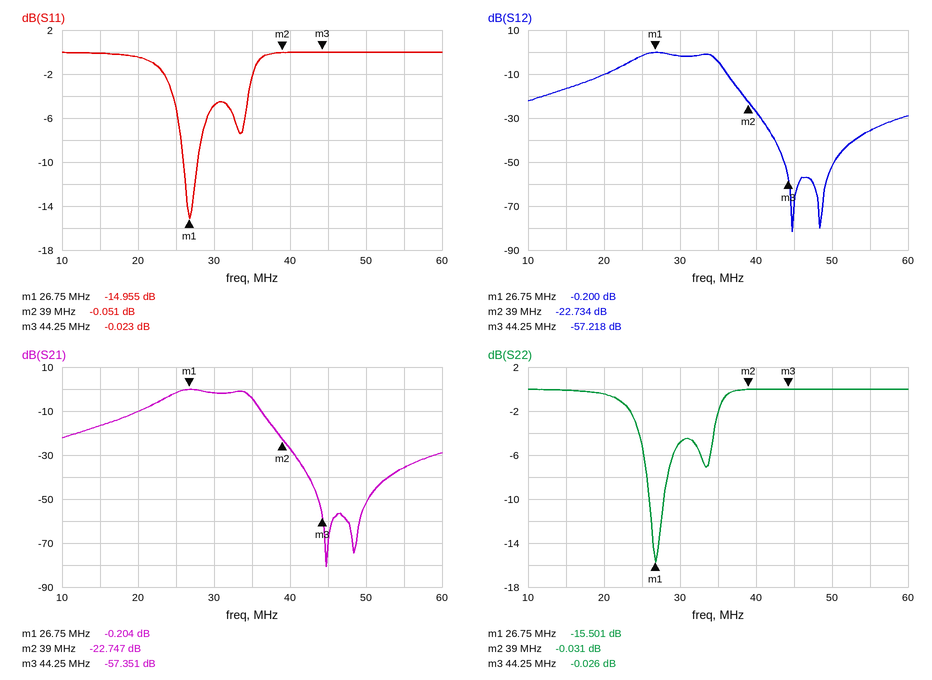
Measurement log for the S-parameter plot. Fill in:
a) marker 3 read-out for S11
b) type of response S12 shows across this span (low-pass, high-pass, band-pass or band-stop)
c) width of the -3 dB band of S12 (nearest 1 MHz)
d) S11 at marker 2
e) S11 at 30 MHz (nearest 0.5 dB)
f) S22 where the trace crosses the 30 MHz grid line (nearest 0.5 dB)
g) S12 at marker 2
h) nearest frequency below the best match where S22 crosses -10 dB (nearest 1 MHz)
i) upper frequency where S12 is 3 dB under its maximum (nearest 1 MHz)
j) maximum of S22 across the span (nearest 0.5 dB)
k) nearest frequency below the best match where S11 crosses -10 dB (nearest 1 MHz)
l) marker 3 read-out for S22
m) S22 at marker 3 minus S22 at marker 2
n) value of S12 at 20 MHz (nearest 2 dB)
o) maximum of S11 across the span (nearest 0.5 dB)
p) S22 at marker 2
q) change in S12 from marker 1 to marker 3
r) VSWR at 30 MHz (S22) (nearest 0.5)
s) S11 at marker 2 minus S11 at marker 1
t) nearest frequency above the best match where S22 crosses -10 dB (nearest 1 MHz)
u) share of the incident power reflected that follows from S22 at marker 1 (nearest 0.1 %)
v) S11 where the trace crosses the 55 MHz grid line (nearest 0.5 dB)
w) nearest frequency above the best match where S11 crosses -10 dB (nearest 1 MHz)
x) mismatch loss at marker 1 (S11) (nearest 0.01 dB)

-0.023 dB
band-pass
11 MHz
-0.051 dB
-5.0 dB
-5.0 dB
-22.734 dB
26 MHz
35 MHz
0.0 dB
26 MHz
-0.026 dB
0.005 dB
-10 dB
0.0 dB
-0.031 dB
-57.018 dB
3.5
14.904 dB
28 MHz
2.8 %
0.0 dB
28 MHz
0.14 dB
